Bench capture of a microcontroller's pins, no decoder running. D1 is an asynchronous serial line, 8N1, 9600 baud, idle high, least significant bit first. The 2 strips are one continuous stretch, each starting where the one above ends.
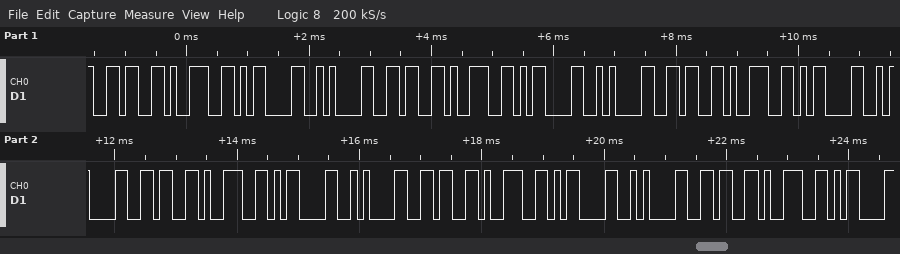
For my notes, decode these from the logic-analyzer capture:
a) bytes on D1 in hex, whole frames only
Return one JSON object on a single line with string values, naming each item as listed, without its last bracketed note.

{"bytes on D1 in hex, whole frames only": "36 39 0D 0A 36 39 0D 0A 36 39 0D 0A 36 39 0D 0A 36 39 0D 0A 36 39 0D"}
